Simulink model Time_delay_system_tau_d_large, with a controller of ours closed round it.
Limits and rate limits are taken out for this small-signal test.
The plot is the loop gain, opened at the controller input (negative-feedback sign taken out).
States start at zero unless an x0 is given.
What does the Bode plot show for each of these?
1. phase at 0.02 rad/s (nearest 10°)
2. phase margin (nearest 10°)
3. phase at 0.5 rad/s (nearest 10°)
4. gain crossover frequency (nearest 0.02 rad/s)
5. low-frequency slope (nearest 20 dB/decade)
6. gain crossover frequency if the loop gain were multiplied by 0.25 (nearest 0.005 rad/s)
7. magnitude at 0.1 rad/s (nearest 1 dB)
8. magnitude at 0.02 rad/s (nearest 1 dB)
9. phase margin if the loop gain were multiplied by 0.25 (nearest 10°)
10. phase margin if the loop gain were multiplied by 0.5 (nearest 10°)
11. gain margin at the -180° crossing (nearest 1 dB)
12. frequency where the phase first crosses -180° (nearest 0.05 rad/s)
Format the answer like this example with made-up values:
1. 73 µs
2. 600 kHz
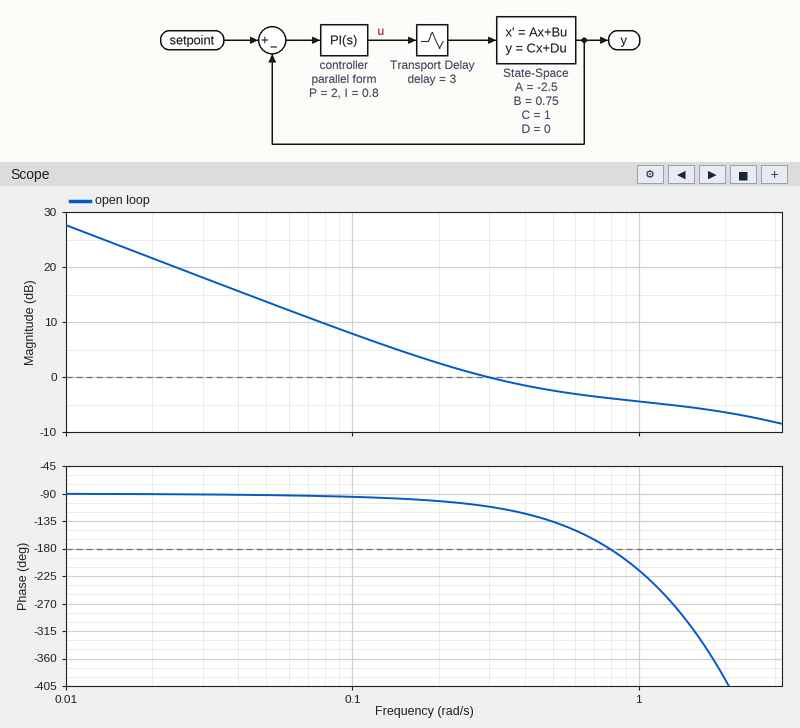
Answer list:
1. -90°
2. 70°
3. -140°
4. 0.30 rad/s
5. -20 dB/decade
6. 0.060 rad/s
7. 8 dB
8. 22 dB
9. 90°
10. 80°
11. 4 dB
12. 0.80 rad/s
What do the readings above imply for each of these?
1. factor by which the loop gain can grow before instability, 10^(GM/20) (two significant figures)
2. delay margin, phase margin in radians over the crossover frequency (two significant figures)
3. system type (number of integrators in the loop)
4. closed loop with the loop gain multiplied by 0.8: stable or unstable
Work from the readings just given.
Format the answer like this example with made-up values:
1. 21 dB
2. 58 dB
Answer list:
1. 1.6
2. 4.1 s
3. 1
4. stable
